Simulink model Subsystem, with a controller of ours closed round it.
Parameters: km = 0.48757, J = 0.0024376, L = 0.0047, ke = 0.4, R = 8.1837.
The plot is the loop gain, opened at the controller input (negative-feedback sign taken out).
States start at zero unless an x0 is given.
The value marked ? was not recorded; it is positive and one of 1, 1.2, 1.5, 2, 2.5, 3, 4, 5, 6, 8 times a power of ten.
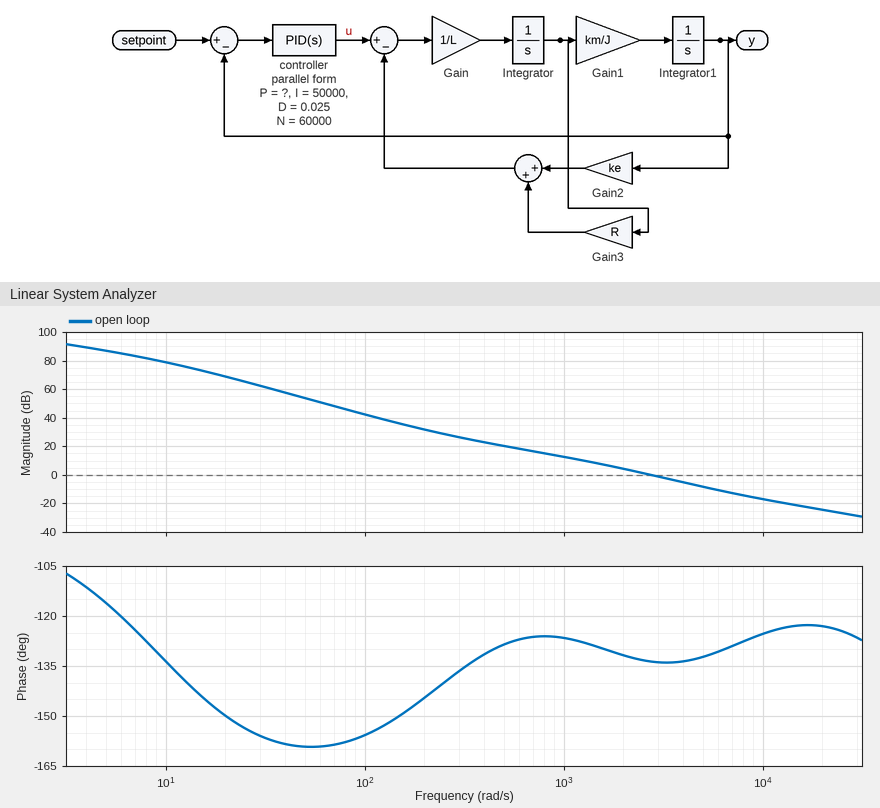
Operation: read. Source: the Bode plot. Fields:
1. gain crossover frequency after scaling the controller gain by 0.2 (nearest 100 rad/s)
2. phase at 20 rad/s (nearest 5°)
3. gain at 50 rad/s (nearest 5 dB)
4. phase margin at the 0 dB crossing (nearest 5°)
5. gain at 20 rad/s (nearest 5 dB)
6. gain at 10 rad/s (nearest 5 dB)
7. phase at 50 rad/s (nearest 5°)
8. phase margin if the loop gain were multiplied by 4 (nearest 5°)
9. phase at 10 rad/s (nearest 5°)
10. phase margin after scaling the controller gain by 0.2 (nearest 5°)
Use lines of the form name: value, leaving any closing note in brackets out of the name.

gain crossover frequency after scaling the controller gain by 0.2: 900 rad/s
phase at 20 rad/s: -150°
gain at 50 rad/s: 55 dB
phase margin at the 0 dB crossing: 45°
gain at 20 rad/s: 70 dB
gain at 10 rad/s: 80 dB
phase at 50 rad/s: -160°
phase margin if the loop gain were multiplied by 4: 50°
phase at 10 rad/s: -135°
phase margin after scaling the controller gain by 0.2: 55°
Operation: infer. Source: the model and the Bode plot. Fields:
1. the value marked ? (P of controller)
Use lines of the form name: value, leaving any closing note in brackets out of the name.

the value marked ?: 200
